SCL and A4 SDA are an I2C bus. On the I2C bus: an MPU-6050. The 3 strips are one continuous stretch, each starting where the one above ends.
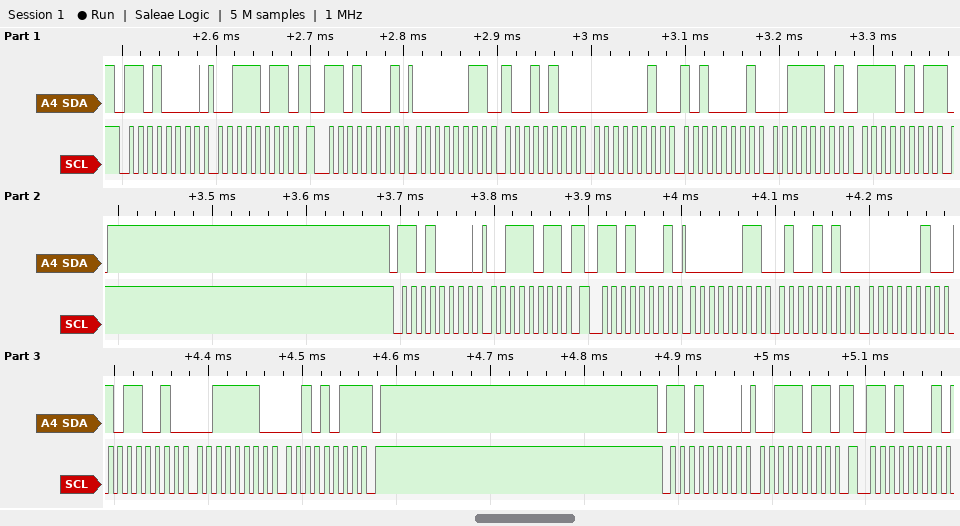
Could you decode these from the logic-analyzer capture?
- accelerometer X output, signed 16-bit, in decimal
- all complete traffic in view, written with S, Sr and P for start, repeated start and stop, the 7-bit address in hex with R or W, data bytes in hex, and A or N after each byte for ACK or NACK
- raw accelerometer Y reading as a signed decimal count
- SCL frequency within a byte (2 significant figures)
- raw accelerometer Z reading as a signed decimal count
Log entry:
916
S 68W A 3B A Sr 68R A 03 A 94 A 02 A A1 A 3D A F5 N P S 68W A 3B A Sr 68R A 03 A 4A A 02 A B2 A 3E A 2B N P S 68W A 3B A Sr 68R A
673
100 kHz
15861
